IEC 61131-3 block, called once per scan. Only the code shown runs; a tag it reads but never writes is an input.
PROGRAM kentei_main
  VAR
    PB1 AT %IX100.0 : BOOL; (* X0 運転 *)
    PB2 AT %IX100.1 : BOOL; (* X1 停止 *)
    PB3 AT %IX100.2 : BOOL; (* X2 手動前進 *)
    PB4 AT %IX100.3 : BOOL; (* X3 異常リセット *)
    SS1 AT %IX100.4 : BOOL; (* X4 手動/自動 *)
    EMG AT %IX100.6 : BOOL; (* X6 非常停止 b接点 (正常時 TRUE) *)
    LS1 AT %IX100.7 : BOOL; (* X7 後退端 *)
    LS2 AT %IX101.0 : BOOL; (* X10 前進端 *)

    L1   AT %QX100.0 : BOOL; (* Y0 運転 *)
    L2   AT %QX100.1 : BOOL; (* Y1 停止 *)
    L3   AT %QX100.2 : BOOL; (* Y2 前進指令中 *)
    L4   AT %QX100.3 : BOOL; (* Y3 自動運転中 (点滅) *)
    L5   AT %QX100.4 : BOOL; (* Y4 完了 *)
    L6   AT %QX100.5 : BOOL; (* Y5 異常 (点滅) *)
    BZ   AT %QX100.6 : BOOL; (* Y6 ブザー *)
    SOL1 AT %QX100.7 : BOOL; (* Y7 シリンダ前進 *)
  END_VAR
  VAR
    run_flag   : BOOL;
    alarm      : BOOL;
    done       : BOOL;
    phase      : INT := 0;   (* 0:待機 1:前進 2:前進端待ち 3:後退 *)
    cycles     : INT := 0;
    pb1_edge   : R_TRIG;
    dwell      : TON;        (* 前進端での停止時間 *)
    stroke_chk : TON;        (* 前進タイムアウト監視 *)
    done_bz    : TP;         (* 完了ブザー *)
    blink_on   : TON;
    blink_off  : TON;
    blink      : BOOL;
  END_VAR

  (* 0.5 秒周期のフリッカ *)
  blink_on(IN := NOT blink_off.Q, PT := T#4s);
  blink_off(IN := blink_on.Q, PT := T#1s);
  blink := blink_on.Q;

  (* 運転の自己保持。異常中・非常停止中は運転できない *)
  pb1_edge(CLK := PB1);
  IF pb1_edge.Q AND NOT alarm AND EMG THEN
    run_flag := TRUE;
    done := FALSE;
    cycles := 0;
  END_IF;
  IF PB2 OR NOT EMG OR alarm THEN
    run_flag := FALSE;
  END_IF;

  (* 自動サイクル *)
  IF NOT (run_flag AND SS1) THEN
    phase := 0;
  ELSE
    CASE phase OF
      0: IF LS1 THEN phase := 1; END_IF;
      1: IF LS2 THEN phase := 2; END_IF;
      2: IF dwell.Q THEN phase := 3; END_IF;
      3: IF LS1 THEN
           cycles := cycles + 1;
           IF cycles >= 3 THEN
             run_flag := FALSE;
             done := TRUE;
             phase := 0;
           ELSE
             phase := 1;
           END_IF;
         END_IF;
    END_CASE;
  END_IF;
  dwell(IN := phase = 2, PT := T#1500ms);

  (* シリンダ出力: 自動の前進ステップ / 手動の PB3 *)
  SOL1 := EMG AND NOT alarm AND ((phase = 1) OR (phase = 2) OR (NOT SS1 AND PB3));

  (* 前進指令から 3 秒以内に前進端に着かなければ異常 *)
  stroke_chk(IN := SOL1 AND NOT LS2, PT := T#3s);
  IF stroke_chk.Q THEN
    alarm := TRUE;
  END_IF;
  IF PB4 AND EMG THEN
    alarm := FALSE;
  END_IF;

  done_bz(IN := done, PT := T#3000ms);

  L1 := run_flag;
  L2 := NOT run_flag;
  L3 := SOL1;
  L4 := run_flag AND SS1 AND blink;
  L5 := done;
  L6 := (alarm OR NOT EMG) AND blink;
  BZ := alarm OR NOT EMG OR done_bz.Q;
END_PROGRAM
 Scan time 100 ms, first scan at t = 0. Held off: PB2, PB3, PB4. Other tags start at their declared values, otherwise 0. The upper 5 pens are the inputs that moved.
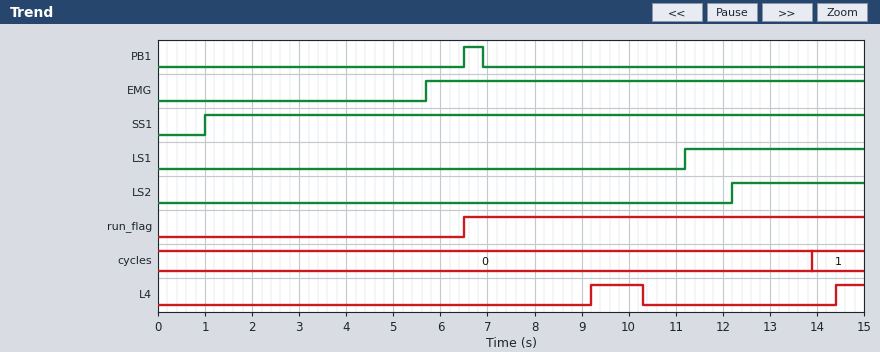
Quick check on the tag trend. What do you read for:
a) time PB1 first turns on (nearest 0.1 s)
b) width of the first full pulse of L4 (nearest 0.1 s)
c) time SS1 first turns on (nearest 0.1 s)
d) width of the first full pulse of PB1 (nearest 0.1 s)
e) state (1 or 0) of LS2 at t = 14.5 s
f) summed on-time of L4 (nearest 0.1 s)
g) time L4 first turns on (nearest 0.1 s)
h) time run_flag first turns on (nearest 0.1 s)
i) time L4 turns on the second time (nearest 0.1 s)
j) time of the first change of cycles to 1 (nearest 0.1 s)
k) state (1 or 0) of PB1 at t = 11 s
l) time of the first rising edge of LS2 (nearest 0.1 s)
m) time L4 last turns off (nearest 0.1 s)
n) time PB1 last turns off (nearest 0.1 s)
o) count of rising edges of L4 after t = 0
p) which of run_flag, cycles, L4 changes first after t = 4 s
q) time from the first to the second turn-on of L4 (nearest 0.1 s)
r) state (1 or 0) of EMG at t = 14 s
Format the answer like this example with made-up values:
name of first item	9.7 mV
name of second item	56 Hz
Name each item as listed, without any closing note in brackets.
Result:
time PB1 first turns on	6.5 s
width of the first full pulse of L4	1.1 s
time SS1 first turns on	1.0 s
width of the first full pulse of PB1	0.4 s
state (1 or 0) of LS2 at t = 14.5 s	1
summed on-time of L4	1.7 s
time L4 first turns on	9.2 s
time run_flag first turns on	6.5 s
time L4 turns on the second time	14.4 s
time of the first change of cycles to 1	13.9 s
state (1 or 0) of PB1 at t = 11 s	0
time of the first rising edge of LS2	12.2 s
time L4 last turns off	10.3 s
time PB1 last turns off	6.9 s
count of rising edges of L4 after t = 0	2
which of run_flag, cycles, L4 changes first after t = 4 s	run_flag
time from the first to the second turn-on of L4	5.2 s
state (1 or 0) of EMG at t = 14 s	1
